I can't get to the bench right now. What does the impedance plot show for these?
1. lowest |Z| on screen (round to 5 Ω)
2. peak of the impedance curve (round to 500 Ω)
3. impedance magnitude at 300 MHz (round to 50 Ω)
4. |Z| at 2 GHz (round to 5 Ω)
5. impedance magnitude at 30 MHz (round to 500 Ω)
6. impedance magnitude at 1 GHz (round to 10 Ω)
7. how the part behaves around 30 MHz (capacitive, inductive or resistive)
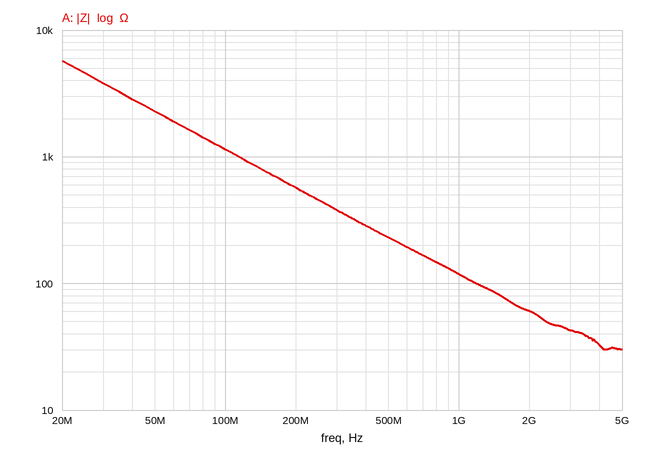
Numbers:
30 Ω
5.5 kΩ
400 Ω
60 Ω
4.0 kΩ
120 Ω
capacitive
